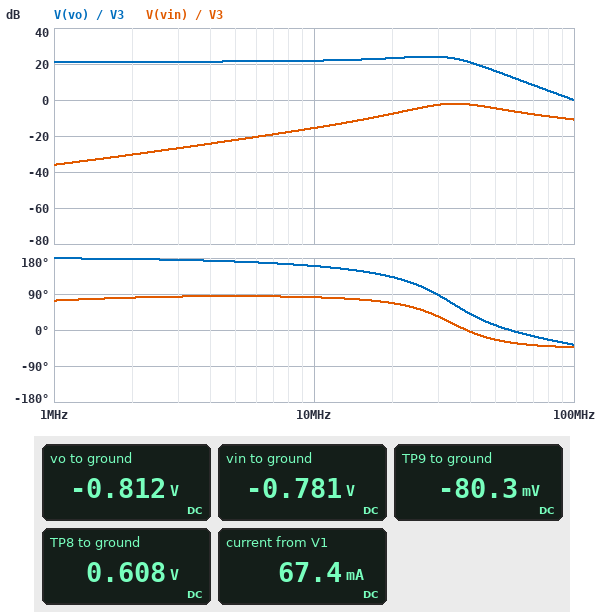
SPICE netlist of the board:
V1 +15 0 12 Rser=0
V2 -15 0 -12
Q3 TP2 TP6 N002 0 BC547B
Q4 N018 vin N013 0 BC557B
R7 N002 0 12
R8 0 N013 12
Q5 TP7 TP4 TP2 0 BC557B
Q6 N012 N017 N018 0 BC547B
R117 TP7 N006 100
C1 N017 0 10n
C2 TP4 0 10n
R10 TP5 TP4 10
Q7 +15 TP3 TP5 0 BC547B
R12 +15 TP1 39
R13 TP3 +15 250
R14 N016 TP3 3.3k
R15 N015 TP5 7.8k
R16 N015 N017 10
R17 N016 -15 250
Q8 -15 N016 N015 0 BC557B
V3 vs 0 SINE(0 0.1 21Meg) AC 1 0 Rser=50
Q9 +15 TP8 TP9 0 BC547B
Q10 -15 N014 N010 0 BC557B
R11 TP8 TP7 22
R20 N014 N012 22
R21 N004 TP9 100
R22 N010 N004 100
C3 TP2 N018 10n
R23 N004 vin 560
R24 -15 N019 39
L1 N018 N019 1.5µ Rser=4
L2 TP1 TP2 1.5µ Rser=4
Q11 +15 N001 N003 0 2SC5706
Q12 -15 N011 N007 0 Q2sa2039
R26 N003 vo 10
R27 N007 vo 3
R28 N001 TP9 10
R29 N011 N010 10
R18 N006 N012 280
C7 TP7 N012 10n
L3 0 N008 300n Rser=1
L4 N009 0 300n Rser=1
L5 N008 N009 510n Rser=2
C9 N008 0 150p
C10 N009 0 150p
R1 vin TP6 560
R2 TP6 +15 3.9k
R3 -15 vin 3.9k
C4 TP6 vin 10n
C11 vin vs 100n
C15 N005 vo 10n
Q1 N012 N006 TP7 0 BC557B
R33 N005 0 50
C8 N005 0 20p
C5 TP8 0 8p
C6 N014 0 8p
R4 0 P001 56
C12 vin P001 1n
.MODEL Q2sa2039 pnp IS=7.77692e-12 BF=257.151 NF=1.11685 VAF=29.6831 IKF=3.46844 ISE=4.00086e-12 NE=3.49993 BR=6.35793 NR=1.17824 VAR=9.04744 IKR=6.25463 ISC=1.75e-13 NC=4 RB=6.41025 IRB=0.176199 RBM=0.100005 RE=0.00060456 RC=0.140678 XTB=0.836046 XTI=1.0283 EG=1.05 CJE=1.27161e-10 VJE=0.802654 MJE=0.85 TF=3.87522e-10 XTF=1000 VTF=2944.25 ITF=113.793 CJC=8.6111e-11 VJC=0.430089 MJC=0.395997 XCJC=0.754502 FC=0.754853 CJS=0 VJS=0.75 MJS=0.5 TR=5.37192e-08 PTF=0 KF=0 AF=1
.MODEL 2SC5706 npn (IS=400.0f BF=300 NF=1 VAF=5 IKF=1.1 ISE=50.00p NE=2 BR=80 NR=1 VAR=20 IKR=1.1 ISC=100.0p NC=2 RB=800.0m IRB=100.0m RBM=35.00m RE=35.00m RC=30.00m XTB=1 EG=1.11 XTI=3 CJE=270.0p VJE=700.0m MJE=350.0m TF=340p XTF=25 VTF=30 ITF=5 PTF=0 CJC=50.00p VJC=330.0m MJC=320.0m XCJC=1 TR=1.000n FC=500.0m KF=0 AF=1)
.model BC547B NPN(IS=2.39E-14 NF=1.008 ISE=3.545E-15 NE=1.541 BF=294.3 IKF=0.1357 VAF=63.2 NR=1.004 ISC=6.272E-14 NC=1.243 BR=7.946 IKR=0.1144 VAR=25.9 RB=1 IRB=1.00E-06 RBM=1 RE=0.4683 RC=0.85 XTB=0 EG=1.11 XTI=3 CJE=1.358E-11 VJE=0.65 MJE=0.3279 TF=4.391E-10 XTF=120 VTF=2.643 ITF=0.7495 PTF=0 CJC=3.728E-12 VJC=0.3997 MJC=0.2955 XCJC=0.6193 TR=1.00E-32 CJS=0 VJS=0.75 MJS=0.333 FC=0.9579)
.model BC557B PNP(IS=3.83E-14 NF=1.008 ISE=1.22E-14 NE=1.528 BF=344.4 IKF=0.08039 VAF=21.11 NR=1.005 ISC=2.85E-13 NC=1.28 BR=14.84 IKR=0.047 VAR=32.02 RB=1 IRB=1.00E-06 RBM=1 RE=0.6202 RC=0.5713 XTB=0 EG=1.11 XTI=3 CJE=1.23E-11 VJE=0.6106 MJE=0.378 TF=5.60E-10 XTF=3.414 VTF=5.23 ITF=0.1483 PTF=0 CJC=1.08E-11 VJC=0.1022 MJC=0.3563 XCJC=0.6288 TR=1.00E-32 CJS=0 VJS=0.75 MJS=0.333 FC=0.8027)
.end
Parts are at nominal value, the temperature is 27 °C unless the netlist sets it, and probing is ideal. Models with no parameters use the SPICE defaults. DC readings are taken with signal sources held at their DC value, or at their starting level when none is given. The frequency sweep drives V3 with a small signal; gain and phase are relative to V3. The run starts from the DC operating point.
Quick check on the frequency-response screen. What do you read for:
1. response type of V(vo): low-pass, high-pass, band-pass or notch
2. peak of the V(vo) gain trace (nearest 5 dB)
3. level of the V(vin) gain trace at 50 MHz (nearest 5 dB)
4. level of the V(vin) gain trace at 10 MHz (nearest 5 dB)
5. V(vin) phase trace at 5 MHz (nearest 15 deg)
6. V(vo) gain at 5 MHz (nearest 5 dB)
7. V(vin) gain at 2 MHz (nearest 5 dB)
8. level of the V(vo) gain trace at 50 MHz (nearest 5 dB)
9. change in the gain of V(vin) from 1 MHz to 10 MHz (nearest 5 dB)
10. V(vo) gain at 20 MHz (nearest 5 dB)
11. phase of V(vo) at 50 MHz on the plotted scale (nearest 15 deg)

low-pass
25 dB
-5 dB
-15 dB
90 deg
20 dB
-30 dB
15 dB
20 dB
25 dB
15 deg
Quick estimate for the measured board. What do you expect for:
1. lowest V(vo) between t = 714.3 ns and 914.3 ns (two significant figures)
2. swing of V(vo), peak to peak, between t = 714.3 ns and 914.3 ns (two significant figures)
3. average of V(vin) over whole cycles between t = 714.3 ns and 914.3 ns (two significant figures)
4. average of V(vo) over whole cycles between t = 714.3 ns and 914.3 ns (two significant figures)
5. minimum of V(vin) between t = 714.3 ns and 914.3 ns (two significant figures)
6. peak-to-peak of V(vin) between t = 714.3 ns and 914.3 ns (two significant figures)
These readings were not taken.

-2.4 V
3.0 V
-780 mV
-820 mV
-830 mV
93 mV
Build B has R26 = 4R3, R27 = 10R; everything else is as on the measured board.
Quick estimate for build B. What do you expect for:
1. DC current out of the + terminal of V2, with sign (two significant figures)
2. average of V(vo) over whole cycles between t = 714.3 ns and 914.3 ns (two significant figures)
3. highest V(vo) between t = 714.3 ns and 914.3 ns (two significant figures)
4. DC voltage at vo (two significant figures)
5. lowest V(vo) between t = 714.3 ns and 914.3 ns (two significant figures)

-66 mA
-710 mV
840 mV
-730 mV
-2.1 V
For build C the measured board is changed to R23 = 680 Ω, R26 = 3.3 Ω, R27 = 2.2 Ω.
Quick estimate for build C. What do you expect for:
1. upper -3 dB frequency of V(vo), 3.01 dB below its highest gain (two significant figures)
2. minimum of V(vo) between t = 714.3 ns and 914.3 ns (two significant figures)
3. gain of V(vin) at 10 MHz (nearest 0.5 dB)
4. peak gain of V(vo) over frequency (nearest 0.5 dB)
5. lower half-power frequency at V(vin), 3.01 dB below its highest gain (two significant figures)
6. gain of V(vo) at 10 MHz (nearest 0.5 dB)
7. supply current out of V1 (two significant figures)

37 MHz
-2.6 V
-14.0 dB
25.0 dB
22 MHz
23.5 dB
79 mA
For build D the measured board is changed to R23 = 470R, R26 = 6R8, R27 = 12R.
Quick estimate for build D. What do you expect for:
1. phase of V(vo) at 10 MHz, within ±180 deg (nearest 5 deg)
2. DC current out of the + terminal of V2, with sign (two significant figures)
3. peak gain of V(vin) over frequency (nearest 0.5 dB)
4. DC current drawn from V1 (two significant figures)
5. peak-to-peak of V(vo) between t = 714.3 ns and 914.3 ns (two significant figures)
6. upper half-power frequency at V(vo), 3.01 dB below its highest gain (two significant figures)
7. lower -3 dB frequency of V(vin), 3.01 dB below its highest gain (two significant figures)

165 deg
-63 mA
-1.5 dB
64 mA
2.5 V
42 MHz
27 MHz
